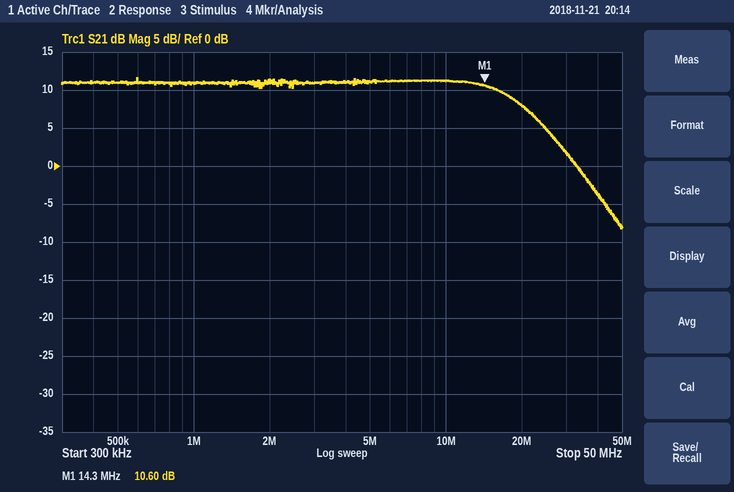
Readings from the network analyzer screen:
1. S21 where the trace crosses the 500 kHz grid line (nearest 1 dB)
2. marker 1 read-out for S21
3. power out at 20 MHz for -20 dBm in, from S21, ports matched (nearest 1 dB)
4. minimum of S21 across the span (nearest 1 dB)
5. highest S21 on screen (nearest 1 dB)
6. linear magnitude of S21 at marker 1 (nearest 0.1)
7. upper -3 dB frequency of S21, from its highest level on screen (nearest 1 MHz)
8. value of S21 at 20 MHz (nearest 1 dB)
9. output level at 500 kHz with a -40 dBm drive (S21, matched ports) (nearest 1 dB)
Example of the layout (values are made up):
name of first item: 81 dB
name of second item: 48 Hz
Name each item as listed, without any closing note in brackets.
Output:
S21 where the trace crosses the 500 kHz grid line: 11 dB
marker 1 read-out for S21: 10.60 dB
power out at 20 MHz for -20 dBm in, from S21, ports matched: -12 dBm
minimum of S21 across the span: -8 dB
highest S21 on screen: 12 dB
linear magnitude of S21 at marker 1: 3.4
upper -3 dB frequency of S21, from its highest level on screen: 19 MHz
value of S21 at 20 MHz: 8 dB
output level at 500 kHz with a -40 dBm drive (S21, matched ports): -29 dBm
